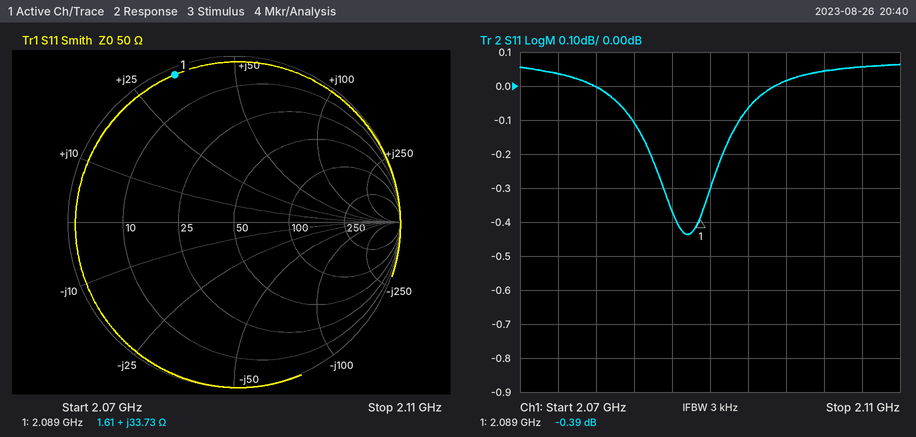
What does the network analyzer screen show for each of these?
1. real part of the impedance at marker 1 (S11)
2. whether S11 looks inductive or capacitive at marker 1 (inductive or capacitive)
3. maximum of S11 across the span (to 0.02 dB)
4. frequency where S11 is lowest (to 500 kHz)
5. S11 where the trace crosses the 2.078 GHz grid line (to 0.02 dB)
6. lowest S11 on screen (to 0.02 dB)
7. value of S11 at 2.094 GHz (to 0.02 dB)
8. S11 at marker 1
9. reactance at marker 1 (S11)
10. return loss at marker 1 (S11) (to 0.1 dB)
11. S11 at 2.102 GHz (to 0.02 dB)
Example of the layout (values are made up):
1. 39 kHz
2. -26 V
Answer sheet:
1. 1.61 Ω
2. inductive
3. 0.06 dB
4. 2.0875 GHz
5. 0.00 dB
6. -0.44 dB
7. -0.06 dB
8. -0.39 dB
9. +33.73 Ω
10. 0.4 dB
11. 0.04 dB
